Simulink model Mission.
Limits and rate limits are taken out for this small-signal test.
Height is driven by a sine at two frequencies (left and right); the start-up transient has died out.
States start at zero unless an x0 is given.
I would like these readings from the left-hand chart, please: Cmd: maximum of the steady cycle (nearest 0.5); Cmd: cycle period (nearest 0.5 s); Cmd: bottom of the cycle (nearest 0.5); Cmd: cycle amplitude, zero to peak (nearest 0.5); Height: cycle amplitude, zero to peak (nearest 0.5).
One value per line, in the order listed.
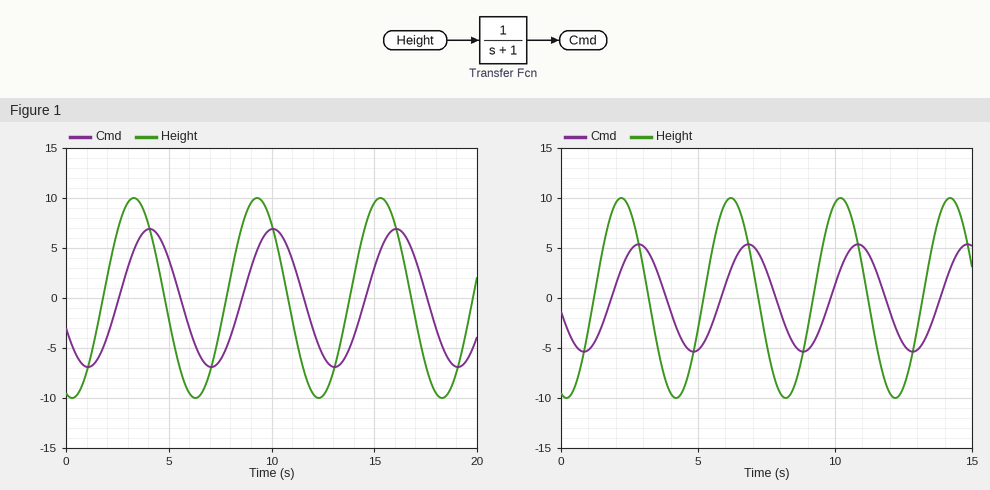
7.0
6.0 s
-7.0
7.0
10.0
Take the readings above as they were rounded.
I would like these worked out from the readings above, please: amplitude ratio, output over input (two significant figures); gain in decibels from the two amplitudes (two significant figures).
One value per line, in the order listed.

0.70
-3.1 dB
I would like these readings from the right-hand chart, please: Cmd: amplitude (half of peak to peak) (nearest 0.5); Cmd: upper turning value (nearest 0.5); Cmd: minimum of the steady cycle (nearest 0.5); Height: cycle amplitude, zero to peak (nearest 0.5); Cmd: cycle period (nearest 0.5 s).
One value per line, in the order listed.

5.5
5.5
-5.5
10.0
4.0 s
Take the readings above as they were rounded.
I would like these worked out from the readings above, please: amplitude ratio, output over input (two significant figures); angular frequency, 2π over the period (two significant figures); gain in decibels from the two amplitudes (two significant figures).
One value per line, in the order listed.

0.55
1.6 rad/s
-5.2 dB
